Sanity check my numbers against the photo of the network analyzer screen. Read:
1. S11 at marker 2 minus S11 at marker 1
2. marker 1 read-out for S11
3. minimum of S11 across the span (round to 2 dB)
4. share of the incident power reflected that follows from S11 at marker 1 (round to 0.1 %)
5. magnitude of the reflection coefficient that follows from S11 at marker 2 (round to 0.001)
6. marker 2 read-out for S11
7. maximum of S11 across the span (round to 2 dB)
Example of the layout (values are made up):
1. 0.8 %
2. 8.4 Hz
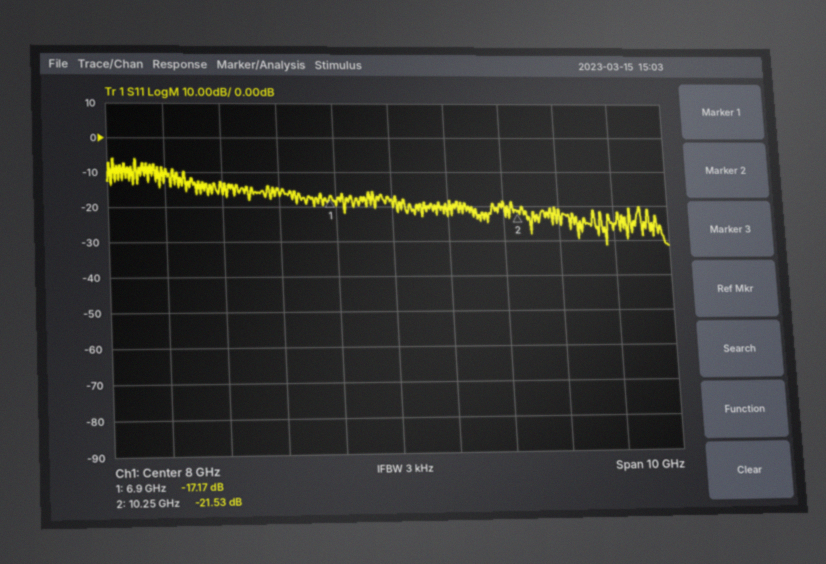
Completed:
1. -4.36 dB
2. -17.17 dB
3. -32 dB
4. 1.9 %
5. 0.084
6. -21.53 dB
7. -6 dB
